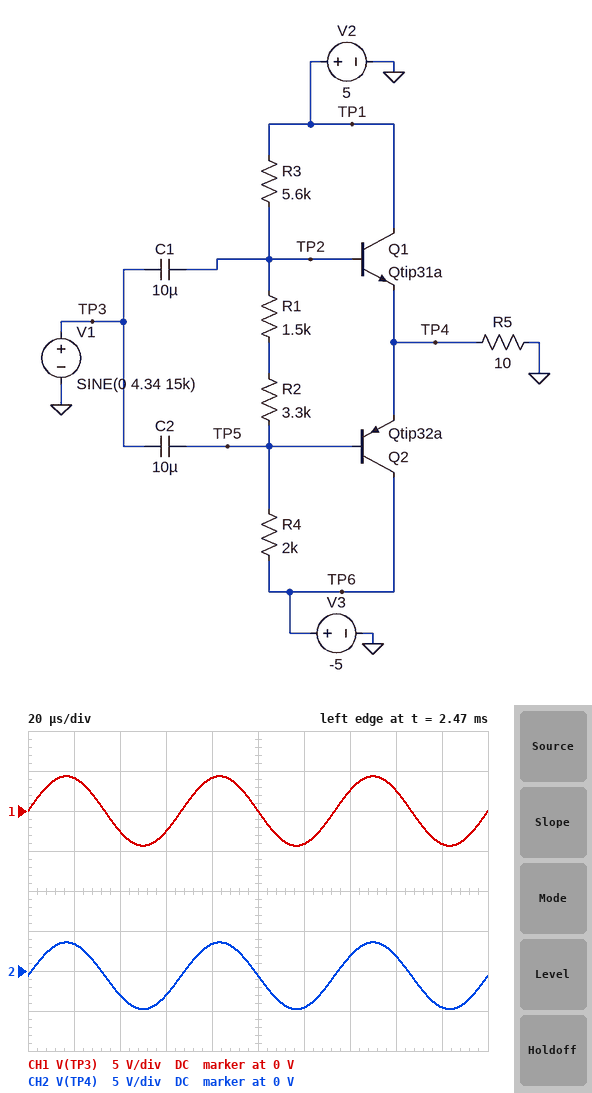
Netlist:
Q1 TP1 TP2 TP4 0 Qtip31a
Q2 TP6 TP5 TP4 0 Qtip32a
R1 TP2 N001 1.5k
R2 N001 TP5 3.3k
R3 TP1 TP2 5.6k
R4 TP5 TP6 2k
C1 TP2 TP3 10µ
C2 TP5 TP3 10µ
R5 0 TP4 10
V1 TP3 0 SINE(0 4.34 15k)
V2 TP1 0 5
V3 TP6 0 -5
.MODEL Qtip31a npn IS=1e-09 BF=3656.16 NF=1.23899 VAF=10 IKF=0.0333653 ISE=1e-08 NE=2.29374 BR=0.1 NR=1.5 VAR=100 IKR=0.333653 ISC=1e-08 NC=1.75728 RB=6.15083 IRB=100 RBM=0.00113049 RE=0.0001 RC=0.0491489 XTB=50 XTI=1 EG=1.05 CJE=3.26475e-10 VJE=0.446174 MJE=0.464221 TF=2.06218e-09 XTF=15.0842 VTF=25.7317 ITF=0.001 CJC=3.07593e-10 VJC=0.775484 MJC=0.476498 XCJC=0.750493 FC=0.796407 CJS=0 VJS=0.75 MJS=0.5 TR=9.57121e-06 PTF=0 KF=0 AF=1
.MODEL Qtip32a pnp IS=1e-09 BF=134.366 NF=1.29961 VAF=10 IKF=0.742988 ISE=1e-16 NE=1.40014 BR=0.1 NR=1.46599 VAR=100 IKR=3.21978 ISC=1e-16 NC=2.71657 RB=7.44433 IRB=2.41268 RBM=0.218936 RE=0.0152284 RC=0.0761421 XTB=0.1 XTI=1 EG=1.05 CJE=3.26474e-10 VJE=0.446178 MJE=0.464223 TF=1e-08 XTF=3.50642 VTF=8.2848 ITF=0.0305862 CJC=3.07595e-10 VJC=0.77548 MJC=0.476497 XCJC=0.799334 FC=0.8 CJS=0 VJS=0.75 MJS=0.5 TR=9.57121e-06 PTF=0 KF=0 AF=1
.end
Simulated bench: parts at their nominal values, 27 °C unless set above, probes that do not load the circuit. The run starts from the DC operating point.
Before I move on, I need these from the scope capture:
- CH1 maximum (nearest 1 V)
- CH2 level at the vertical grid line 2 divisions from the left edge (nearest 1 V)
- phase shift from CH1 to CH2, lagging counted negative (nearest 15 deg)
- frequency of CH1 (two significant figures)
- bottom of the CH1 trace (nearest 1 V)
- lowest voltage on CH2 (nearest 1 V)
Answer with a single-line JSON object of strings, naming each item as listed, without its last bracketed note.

{"CH1 maximum": "4 V", "CH2 level at the vertical grid line 2 divisions from the left edge": "-3 V", "phase shift from CH1 to CH2, lagging counted negative": "0 deg", "frequency of CH1": "15 kHz", "bottom of the CH1 trace": "-4 V", "lowest voltage on CH2": "-5 V"}
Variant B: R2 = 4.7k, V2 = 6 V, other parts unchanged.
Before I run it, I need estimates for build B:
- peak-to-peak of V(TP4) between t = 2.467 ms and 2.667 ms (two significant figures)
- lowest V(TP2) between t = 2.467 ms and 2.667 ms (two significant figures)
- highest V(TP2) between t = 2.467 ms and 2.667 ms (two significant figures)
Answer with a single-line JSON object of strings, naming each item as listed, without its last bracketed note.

{"peak-to-peak of V(TP4) between t = 2.467 ms and 2.667 ms": "8.5 V", "lowest V(TP2) between t = 2.467 ms and 2.667 ms": "-4.1 V", "highest V(TP2) between t = 2.467 ms and 2.667 ms": "4.6 V"}
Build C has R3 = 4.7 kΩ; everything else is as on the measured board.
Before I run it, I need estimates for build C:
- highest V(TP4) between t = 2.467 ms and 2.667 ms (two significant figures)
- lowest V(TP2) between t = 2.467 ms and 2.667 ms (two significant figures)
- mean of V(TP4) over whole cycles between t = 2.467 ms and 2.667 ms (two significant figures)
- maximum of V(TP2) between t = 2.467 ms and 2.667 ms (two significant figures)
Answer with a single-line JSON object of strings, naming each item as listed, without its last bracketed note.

{"highest V(TP4) between t = 2.467 ms and 2.667 ms": "3.7 V", "lowest V(TP2) between t = 2.467 ms and 2.667 ms": "-4.2 V", "mean of V(TP4) over whole cycles between t = 2.467 ms and 2.667 ms": "-470 mV", "maximum of V(TP2) between t = 2.467 ms and 2.667 ms": "4.5 V"}
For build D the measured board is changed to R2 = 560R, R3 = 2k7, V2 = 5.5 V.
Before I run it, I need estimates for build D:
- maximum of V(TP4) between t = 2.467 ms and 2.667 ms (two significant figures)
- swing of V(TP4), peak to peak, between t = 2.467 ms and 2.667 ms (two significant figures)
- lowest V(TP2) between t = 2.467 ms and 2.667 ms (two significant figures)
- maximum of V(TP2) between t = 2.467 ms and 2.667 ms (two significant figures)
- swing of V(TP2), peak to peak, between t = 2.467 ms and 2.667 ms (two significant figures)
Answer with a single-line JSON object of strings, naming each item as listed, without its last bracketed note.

{"maximum of V(TP4) between t = 2.467 ms and 2.667 ms": "4.4 V", "swing of V(TP4), peak to peak, between t = 2.467 ms and 2.667 ms": "8.5 V", "lowest V(TP2) between t = 2.467 ms and 2.667 ms": "-3.6 V", "maximum of V(TP2) between t = 2.467 ms and 2.667 ms": "5.1 V", "swing of V(TP2), peak to peak, between t = 2.467 ms and 2.667 ms": "8.7 V"}
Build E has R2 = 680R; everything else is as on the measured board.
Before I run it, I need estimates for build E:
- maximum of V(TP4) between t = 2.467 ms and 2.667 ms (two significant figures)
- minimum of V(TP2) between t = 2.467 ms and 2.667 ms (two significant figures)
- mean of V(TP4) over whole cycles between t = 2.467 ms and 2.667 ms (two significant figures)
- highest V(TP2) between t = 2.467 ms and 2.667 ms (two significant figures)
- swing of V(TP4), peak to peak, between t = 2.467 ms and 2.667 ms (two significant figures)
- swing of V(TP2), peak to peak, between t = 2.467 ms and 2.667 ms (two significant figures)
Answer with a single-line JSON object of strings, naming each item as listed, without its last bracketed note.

{"maximum of V(TP4) between t = 2.467 ms and 2.667 ms": "3.4 V", "minimum of V(TP2) between t = 2.467 ms and 2.667 ms": "-4.6 V", "mean of V(TP4) over whole cycles between t = 2.467 ms and 2.667 ms": "-680 mV", "highest V(TP2) between t = 2.467 ms and 2.667 ms": "4.1 V", "swing of V(TP4), peak to peak, between t = 2.467 ms and 2.667 ms": "8.1 V", "swing of V(TP2), peak to peak, between t = 2.467 ms and 2.667 ms": "8.7 V"}
